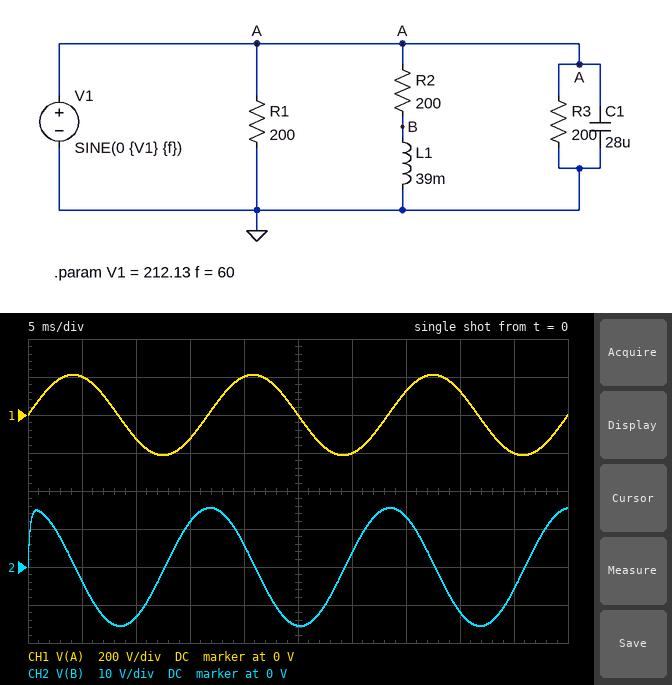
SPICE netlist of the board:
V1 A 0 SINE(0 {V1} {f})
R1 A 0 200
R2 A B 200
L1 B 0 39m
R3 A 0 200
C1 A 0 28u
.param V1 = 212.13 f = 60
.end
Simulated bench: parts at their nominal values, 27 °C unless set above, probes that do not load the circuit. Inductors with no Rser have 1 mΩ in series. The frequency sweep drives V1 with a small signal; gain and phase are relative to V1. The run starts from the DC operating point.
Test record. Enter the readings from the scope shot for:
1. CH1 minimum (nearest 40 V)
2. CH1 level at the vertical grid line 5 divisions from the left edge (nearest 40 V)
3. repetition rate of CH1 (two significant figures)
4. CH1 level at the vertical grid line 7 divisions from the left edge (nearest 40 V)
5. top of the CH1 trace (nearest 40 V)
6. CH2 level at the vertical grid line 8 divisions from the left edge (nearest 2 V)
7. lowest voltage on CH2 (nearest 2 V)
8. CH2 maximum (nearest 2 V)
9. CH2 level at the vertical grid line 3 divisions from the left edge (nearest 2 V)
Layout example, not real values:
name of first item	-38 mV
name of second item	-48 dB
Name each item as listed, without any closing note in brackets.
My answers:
CH1 minimum	-200 V
CH1 level at the vertical grid line 5 divisions from the left edge	0 V
repetition rate of CH1	60 Hz
CH1 level at the vertical grid line 7 divisions from the left edge	120 V
top of the CH1 trace	200 V
CH2 level at the vertical grid line 8 divisions from the left edge	-12 V
lowest voltage on CH2	-16 V
CH2 maximum	16 V
CH2 level at the vertical grid line 3 divisions from the left edge	12 V
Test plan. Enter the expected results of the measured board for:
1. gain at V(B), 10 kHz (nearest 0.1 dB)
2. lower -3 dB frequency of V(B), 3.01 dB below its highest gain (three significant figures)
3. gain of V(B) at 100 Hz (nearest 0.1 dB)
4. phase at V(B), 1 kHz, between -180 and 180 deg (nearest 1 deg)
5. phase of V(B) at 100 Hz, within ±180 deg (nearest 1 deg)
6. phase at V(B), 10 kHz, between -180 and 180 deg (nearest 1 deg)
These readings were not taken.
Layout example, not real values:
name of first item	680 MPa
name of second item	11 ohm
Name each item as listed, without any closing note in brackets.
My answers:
gain at V(B), 10 kHz	0 dB
lower -3 dB frequency of V(B), 3.01 dB below its highest gain	816 Hz
gain of V(B) at 100 Hz	-18.3 dB
phase at V(B), 1 kHz, between -180 and 180 deg	39 deg
phase of V(B) at 100 Hz, within ±180 deg	83 deg
phase at V(B), 10 kHz, between -180 and 180 deg	5 deg
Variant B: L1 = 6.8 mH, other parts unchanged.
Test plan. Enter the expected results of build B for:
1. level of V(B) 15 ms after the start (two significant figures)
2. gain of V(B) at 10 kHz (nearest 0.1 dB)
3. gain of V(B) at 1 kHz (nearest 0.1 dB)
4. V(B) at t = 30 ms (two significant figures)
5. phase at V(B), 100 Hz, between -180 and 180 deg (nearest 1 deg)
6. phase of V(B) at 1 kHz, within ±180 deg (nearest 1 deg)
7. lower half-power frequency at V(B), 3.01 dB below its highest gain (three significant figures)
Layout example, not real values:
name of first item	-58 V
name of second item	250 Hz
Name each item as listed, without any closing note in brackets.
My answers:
level of V(B) 15 ms after the start	2.2 V
gain of V(B) at 10 kHz	-0.9 dB
gain of V(B) at 1 kHz	-13.6 dB
V(B) at t = 30 ms	810 mV
phase at V(B), 100 Hz, between -180 and 180 deg	89 deg
phase of V(B) at 1 kHz, within ±180 deg	78 deg
lower half-power frequency at V(B), 3.01 dB below its highest gain	4.68 kHz
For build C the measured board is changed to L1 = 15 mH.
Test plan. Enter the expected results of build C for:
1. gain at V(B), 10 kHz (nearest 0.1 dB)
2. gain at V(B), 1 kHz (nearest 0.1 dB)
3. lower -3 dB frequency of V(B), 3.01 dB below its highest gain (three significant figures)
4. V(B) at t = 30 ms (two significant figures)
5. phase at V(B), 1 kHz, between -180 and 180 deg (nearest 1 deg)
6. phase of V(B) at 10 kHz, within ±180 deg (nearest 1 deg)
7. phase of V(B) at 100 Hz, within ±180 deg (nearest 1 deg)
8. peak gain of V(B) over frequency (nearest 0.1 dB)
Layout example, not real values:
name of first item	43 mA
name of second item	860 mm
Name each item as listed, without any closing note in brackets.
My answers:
gain at V(B), 10 kHz	-0.2 dB
gain at V(B), 1 kHz	-7.4 dB
lower -3 dB frequency of V(B), 3.01 dB below its highest gain	2.12 kHz
V(B) at t = 30 ms	1.7 V
phase at V(B), 1 kHz, between -180 and 180 deg	65 deg
phase of V(B) at 10 kHz, within ±180 deg	12 deg
phase of V(B) at 100 Hz, within ±180 deg	87 deg
peak gain of V(B) over frequency	0 dB
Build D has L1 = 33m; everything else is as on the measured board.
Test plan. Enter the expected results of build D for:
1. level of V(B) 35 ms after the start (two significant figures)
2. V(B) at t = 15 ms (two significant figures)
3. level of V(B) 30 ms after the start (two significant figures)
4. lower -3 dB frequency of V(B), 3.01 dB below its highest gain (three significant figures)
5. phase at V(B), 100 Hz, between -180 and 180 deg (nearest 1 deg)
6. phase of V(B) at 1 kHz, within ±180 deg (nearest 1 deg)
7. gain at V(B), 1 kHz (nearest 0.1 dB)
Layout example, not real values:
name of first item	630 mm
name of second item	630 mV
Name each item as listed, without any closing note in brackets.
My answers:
level of V(B) 35 ms after the start	11 V
V(B) at t = 15 ms	10 V
level of V(B) 30 ms after the start	3.3 V
lower -3 dB frequency of V(B), 3.01 dB below its highest gain	965 Hz
phase at V(B), 100 Hz, between -180 and 180 deg	84 deg
phase of V(B) at 1 kHz, within ±180 deg	44 deg
gain at V(B), 1 kHz	-2.9 dB
